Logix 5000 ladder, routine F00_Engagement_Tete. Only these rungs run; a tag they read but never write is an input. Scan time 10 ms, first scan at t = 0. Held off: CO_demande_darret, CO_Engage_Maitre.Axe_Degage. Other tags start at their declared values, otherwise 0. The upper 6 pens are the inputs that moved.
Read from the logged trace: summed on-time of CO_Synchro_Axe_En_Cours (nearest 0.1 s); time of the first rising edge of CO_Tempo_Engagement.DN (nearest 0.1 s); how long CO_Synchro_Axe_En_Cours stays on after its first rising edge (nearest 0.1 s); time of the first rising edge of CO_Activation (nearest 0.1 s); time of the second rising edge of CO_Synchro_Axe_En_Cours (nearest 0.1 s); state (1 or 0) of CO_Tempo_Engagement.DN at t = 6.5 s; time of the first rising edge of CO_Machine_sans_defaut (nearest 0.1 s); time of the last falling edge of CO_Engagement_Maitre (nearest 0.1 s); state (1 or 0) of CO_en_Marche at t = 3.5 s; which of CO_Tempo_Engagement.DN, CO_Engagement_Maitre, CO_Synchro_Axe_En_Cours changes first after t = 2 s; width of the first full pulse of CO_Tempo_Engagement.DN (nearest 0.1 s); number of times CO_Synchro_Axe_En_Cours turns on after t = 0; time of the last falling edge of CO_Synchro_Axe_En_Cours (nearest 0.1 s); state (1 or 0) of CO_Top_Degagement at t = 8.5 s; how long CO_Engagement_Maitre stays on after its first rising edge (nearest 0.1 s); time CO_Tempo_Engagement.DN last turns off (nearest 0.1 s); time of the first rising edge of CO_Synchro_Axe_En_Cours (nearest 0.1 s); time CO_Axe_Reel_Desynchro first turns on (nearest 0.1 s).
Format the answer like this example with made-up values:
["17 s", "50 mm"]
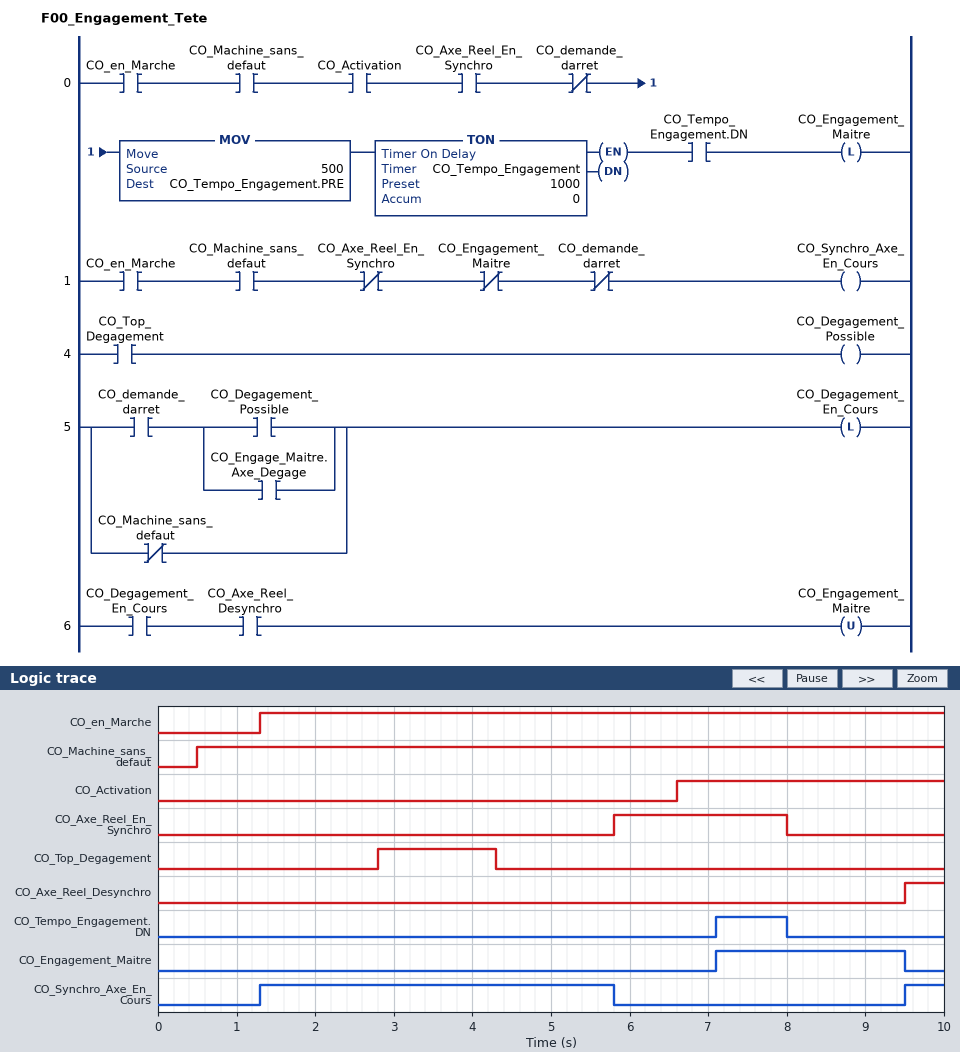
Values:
["5.0 s", "7.1 s", "4.5 s", "6.6 s", "9.5 s", "0", "0.5 s", "9.5 s", "1", "CO_Synchro_Axe_En_Cours", "0.9 s", "2", "5.8 s", "0", "2.4 s", "8.0 s", "1.3 s", "9.5 s"]
